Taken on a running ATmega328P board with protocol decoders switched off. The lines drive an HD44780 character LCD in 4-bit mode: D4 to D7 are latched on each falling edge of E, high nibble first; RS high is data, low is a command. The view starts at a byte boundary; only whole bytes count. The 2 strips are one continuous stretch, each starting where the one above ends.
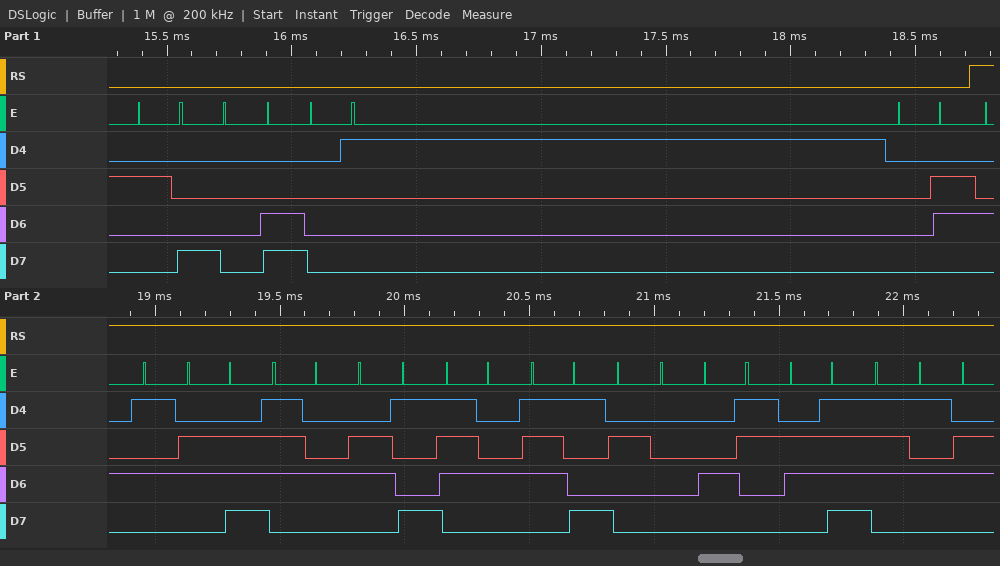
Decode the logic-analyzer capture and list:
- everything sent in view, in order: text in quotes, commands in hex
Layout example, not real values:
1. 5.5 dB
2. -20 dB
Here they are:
1. 0x28 0x0C 0x01 0x06 "Entity Cou"
